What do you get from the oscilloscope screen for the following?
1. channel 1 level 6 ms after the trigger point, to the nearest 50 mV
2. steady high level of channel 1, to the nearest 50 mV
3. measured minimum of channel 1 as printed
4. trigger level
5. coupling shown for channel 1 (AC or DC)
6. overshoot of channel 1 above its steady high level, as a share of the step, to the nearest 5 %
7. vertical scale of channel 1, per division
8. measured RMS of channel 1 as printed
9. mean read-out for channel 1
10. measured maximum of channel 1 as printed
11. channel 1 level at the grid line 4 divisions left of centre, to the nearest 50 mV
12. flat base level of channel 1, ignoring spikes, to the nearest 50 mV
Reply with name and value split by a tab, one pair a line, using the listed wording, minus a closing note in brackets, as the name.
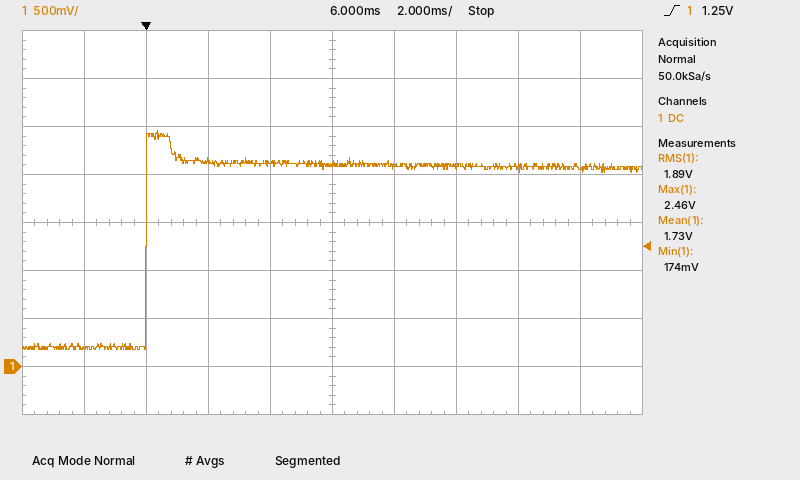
channel 1 level 6 ms after the trigger point, to the nearest 50 mV	2.10 V
steady high level of channel 1, to the nearest 50 mV	2.10 V
measured minimum of channel 1 as printed	174 mV
trigger level	1.25 V
coupling shown for channel 1	DC
overshoot of channel 1 above its steady high level, as a share of the step, to the nearest 5 %	20 %
vertical scale of channel 1, per division	500 mV
measured RMS of channel 1 as printed	1.89 V
mean read-out for channel 1	1.73 V
measured maximum of channel 1 as printed	2.46 V
channel 1 level at the grid line 4 divisions left of centre, to the nearest 50 mV	200 mV
flat base level of channel 1, ignoring spikes, to the nearest 50 mV	200 mV
